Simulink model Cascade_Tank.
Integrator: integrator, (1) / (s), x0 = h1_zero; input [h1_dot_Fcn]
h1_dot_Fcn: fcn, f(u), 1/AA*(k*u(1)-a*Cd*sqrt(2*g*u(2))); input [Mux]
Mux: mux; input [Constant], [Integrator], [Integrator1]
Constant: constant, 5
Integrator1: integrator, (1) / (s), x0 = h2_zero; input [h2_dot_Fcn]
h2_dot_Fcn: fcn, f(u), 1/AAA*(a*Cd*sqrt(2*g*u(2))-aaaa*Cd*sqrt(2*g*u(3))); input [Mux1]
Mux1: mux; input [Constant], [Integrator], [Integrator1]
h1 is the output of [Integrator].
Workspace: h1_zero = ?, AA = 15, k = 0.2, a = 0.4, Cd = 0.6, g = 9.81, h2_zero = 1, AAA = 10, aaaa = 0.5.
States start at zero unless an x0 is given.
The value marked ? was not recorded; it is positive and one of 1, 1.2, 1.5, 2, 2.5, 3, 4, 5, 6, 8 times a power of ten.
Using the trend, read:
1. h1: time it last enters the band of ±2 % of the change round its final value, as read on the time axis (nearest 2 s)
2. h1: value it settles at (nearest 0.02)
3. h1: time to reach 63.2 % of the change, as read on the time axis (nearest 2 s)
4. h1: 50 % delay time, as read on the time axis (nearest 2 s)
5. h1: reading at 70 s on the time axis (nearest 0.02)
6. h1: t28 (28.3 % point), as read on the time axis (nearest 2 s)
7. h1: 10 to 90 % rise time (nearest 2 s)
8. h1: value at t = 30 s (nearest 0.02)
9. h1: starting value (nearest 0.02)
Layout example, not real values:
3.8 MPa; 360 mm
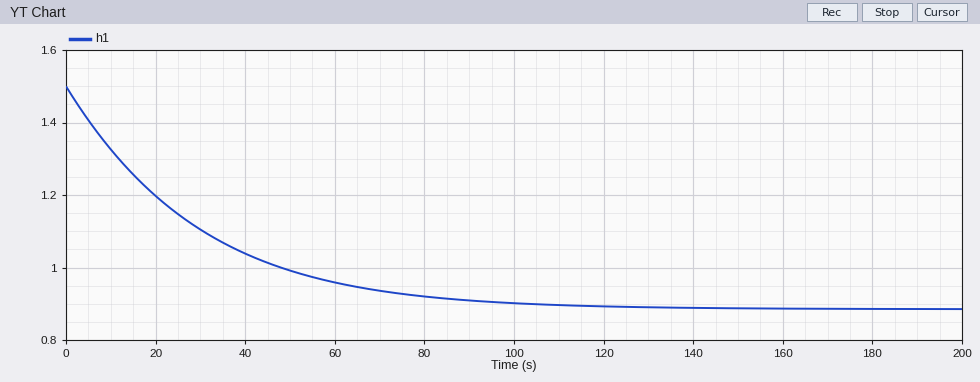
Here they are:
108 s; 0.88; 30 s; 20 s; 0.94; 10 s; 62 s; 1.10; 1.50
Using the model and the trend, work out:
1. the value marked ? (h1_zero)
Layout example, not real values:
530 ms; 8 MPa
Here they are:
1.5
